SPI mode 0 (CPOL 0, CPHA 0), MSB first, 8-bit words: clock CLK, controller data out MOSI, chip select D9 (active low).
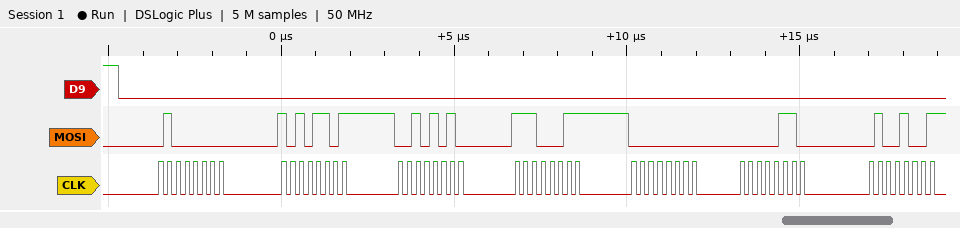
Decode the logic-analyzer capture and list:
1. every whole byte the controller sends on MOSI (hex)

40 AD 2A E3 00 06 49
